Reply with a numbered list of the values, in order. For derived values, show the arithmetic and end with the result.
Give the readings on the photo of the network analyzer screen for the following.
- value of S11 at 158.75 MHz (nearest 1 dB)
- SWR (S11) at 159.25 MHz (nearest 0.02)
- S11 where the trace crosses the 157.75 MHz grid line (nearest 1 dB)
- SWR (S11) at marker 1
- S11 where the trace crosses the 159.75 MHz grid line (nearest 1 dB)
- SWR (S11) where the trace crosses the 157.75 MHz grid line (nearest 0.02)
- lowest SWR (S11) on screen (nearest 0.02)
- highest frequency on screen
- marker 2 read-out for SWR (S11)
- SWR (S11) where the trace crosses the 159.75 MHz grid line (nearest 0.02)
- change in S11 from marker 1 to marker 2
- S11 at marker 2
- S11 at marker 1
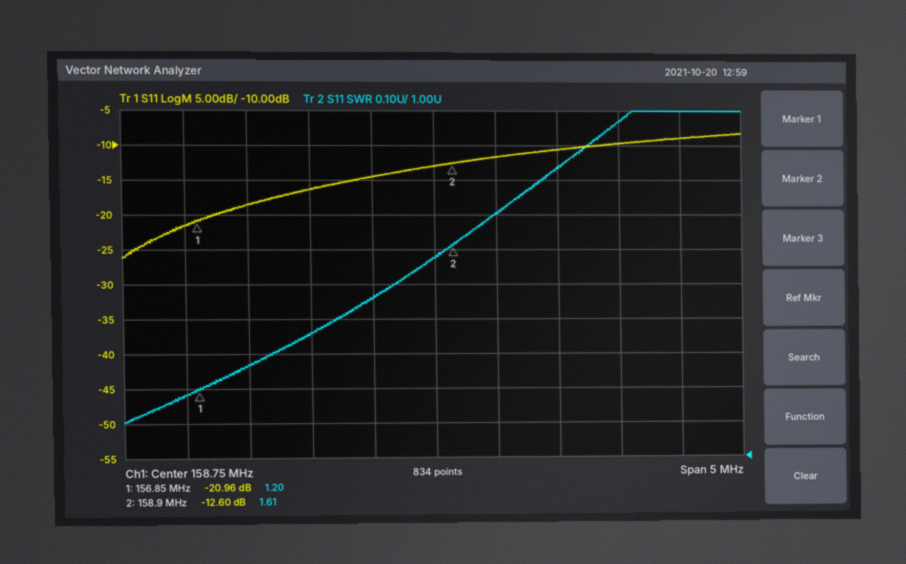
1. -13 dB
2. 1.70
3. -16 dB
4. 1.20
5. -11 dB
6. 1.36
7. 1.10
8. 161.25 MHz
9. 1.61
10. 1.84
11. -12.6 − (-20.96) = 8.36 dB
12. -12.60 dB
13. -20.96 dB
